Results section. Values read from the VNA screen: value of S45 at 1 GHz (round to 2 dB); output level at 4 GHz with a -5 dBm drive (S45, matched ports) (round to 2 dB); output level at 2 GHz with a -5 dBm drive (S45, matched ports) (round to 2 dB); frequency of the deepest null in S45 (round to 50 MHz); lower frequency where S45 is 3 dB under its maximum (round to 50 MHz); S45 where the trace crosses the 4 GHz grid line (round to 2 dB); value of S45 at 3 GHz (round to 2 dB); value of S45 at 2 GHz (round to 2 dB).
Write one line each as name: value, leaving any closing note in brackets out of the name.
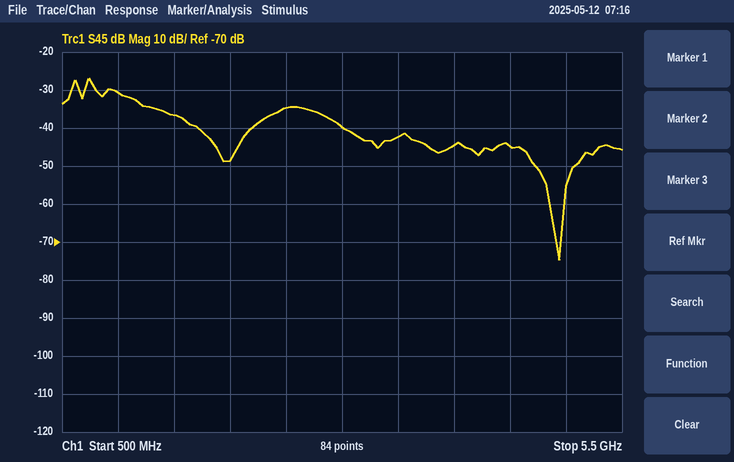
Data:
value of S45 at 1 GHz: -30 dB
output level at 4 GHz with a -5 dBm drive (S45, matched ports): -50 dBm
output level at 2 GHz with a -5 dBm drive (S45, matched ports): -54 dBm
frequency of the deepest null in S45: 4.95 GHz
lower frequency where S45 is 3 dB under its maximum: 700 MHz
S45 where the trace crosses the 4 GHz grid line: -44 dB
value of S45 at 3 GHz: -40 dB
value of S45 at 2 GHz: -48 dB
